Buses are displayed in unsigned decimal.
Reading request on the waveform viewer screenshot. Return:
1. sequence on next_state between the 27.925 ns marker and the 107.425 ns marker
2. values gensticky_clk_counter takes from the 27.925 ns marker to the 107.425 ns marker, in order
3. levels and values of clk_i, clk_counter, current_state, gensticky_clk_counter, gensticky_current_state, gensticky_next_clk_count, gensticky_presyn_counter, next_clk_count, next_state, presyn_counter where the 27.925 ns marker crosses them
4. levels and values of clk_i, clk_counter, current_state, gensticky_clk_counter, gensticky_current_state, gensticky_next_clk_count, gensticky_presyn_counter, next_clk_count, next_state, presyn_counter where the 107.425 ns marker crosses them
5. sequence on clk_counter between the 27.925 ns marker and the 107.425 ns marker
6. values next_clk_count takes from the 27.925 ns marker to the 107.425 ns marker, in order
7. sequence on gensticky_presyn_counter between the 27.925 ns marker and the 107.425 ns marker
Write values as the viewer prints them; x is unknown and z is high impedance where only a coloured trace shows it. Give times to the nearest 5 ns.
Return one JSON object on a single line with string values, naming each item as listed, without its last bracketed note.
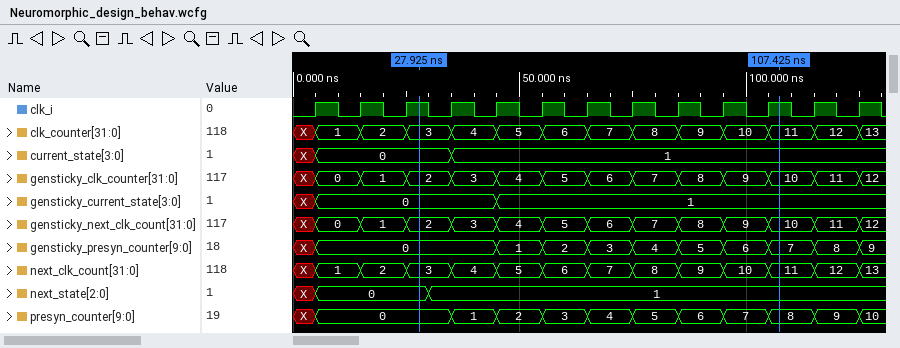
{"sequence on next_state between the 27.925 ns marker and the 107.425 ns marker": "0, 1", "values gensticky_clk_counter takes from the 27.925 ns marker to the 107.425 ns marker, in order": "2, 3, 4, 5, 6, 7, 8, 9, 10", "levels and values of clk_i, clk_counter, current_state, gensticky_clk_counter, gensticky_current_state, gensticky_next_clk_count, gensticky_presyn_counter, next_clk_count, next_state, presyn_counter where the 27.925 ns marker crosses them": "clk_i=1, clk_counter=3, current_state=0, gensticky_clk_counter=2, gensticky_current_state=0, gensticky_next_clk_count=2, gensticky_presyn_counter=0, next_clk_count=3, next_state=0, presyn_counter=0", "levels and values of clk_i, clk_counter, current_state, gensticky_clk_counter, gensticky_current_state, gensticky_next_clk_count, gensticky_presyn_counter, next_clk_count, next_state, presyn_counter where the 107.425 ns marker crosses them": "clk_i=1, clk_counter=11, current_state=1, gensticky_clk_counter=10, gensticky_current_state=1, gensticky_next_clk_count=10, gensticky_presyn_counter=7, next_clk_count=11, next_state=1, presyn_counter=8", "sequence on clk_counter between the 27.925 ns marker and the 107.425 ns marker": "3, 4, 5, 6, 7, 8, 9, 10, 11", "values next_clk_count takes from the 27.925 ns marker to the 107.425 ns marker, in order": "3, 4, 5, 6, 7, 8, 9, 10, 11", "sequence on gensticky_presyn_counter between the 27.925 ns marker and the 107.425 ns marker": "0, 1, 2, 3, 4, 5, 6, 7"}
